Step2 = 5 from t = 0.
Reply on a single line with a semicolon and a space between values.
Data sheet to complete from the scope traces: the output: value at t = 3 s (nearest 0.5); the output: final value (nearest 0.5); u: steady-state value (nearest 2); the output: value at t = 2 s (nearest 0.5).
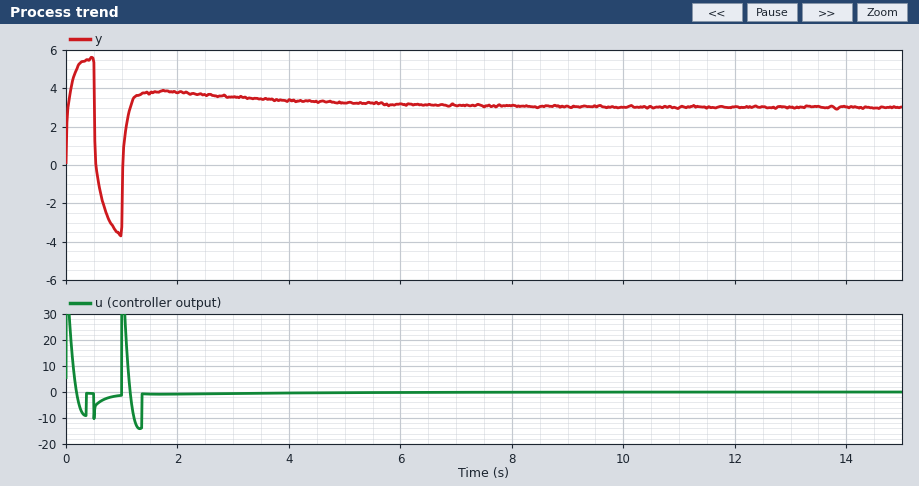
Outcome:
3.5; 3.0; 0; 4.0
